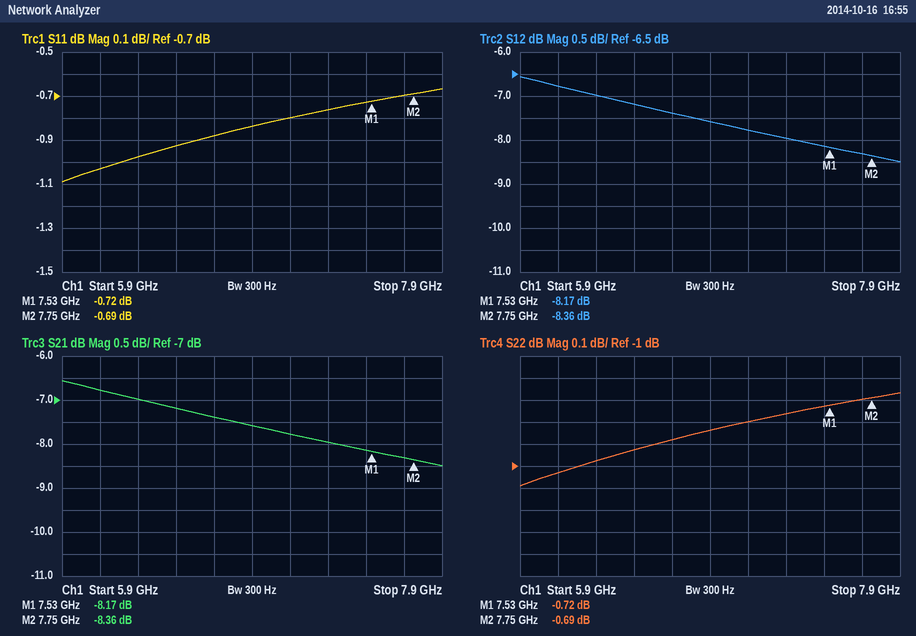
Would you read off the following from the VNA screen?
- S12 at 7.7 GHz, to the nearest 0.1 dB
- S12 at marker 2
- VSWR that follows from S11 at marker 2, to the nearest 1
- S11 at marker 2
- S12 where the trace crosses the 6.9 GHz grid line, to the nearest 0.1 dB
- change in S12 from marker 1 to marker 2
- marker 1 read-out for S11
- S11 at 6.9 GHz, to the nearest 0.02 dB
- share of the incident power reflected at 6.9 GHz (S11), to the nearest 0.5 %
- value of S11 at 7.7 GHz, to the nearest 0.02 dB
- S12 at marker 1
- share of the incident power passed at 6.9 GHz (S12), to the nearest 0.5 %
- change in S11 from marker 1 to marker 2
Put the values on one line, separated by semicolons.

-8.3 dB; -8.36 dB; 25; -0.69 dB; -7.6 dB; -0.19 dB; -0.72 dB; -0.84 dB; 82.5 %; -0.70 dB; -8.17 dB; 17.5 %; 0.03 dB
